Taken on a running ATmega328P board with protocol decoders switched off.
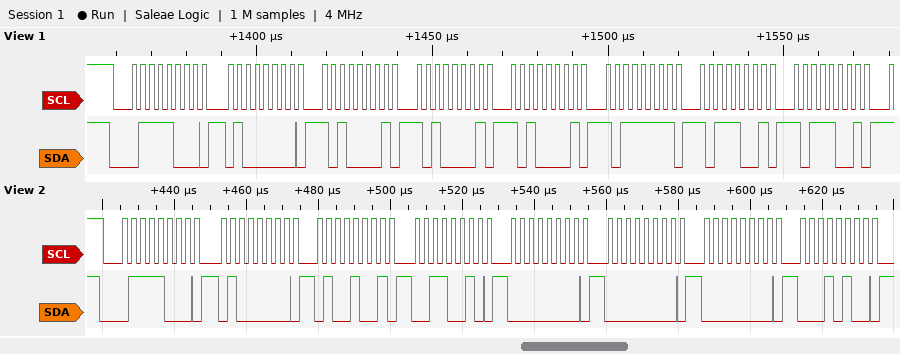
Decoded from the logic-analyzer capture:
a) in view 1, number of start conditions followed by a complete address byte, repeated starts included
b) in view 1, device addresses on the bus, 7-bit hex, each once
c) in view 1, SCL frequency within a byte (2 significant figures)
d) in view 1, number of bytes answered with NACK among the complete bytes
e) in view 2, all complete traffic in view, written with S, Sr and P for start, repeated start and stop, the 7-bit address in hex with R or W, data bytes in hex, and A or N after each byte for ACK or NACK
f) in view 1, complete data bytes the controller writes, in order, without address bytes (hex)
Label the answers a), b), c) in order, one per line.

a) 1
b) 0x3C
c) 400 kHz
d) 0
e) S 3CW A 40 A 49 A 32 A 00 A 00 A 00 A 14 A
f) 40 A1 A1 A1 BF B9 B9
